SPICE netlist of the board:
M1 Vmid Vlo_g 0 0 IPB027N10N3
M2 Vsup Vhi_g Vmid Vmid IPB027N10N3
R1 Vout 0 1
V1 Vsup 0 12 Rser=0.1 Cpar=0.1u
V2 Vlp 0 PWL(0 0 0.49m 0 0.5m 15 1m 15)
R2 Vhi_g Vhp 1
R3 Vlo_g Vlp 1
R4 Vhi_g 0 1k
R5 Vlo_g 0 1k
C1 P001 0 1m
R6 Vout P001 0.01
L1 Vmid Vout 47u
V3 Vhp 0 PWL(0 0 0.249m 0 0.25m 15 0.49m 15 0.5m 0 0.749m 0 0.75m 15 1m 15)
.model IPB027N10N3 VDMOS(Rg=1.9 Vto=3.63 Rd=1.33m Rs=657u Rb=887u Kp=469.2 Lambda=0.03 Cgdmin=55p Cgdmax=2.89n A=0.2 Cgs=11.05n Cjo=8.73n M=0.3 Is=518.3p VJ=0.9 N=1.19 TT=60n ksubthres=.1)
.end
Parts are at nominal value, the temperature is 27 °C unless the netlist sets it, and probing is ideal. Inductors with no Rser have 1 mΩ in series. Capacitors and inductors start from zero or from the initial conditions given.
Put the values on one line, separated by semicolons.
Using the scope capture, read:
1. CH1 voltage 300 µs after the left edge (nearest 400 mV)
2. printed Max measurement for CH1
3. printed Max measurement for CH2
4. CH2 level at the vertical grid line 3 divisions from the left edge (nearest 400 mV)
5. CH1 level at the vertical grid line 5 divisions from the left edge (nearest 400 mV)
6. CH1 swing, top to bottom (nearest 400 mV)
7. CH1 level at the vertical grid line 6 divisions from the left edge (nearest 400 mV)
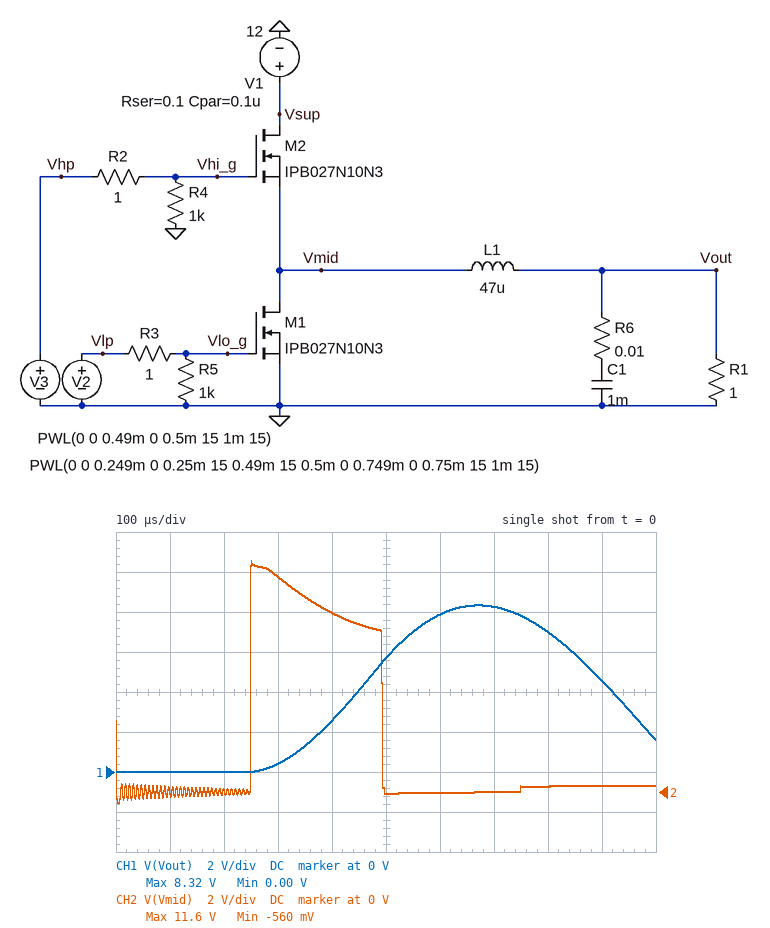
400 mV; 8.32 V; 11.6 V; 10.8 V; 5.6 V; 8.4 V; 8.0 V
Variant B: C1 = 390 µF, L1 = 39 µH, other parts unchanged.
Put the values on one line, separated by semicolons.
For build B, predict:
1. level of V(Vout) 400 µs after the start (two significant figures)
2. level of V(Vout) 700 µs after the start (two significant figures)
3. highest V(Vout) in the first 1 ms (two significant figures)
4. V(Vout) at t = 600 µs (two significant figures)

6.2 V; 4.9 V; 12 V; 11 V
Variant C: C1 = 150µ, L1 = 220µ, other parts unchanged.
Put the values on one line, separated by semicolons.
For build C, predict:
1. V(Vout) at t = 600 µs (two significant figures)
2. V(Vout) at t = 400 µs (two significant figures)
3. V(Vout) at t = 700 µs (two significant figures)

6.9 V; 2.7 V; 6.0 V
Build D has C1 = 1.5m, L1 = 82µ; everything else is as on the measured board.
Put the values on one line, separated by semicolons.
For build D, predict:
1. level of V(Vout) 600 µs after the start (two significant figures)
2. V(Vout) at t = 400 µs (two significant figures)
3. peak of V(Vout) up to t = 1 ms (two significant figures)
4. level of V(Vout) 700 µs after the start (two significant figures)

4.1 V; 1.1 V; 5.7 V; 5.1 V
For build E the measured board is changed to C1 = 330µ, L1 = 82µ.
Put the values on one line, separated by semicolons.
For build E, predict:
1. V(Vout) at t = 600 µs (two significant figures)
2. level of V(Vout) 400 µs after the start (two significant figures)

9.9 V; 3.8 V
